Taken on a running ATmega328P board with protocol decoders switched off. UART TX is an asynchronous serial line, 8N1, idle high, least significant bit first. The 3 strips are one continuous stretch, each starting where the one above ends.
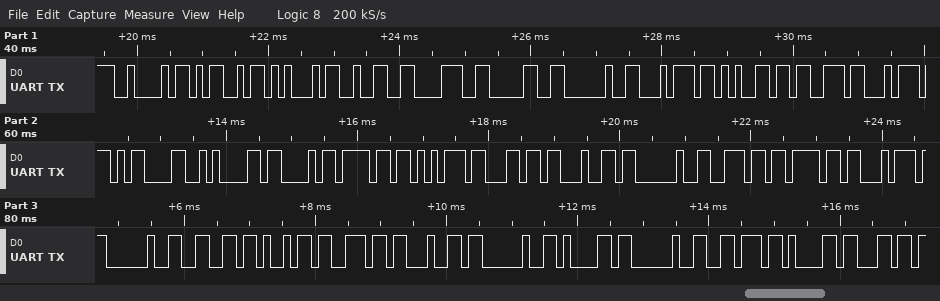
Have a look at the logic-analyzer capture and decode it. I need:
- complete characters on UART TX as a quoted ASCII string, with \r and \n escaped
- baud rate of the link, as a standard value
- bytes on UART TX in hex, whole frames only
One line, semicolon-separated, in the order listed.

"BME280 test\r\nCould not find a val"; 9600 baud; 42 4D 45 32 38 30 20 74 65 73 74 0D 0A 43 6F 75 6C 64 20 6E 6F 74 20 66 69 6E 64 20 61 20 76 61 6C
